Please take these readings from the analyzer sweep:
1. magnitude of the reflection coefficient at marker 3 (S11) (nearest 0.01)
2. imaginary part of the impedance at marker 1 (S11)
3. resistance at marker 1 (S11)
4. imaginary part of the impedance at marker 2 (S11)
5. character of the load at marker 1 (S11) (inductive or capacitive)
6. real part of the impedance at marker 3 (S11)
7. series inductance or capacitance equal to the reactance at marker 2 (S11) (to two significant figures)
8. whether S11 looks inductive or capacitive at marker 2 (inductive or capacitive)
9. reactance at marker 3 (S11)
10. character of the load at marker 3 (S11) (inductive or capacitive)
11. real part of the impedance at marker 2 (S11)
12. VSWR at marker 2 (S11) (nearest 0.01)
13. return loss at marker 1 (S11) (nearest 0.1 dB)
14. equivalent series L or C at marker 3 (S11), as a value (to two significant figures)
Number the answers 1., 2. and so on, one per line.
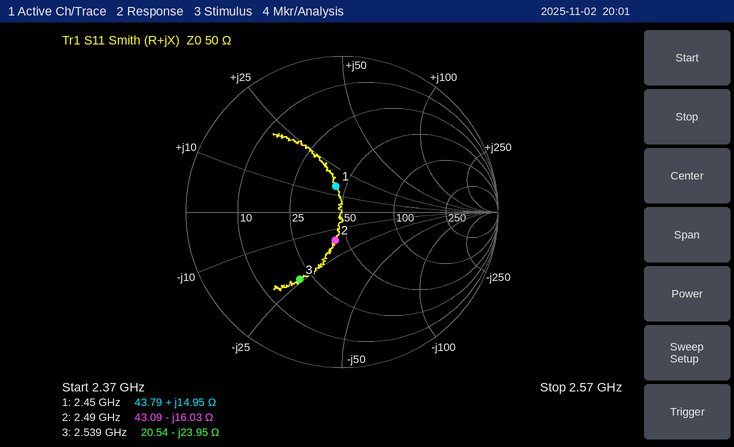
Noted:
1. 0.51
2. +14.95 Ω
3. 43.79 Ω
4. -16.03 Ω
5. inductive
6. 20.54 Ω
7. 4.0 pF
8. capacitive
9. -23.95 Ω
10. capacitive
11. 43.09 Ω
12. 1.45
13. 15.4 dB
14. 2.6 pF
